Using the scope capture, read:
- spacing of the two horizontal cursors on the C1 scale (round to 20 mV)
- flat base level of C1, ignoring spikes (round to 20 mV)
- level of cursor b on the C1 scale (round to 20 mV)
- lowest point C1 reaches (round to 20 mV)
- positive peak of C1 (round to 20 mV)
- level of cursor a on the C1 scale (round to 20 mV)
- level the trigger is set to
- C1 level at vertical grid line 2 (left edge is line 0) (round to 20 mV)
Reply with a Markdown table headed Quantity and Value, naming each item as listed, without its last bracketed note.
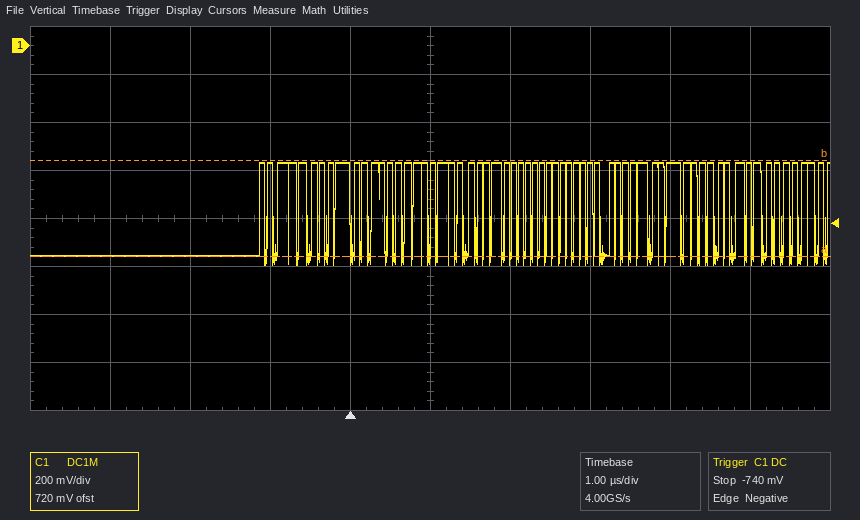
| Quantity | Value |
|---|---|
| spacing of the two horizontal cursors on the C1 scale | 400 mV |
| flat base level of C1, ignoring spikes | -880 mV |
| level of cursor b on the C1 scale | -480 mV |
| lowest point C1 reaches | -920 mV |
| positive peak of C1 | -480 mV |
| level of cursor a on the C1 scale | -880 mV |
| level the trigger is set to | -740 mV |
| C1 level at vertical grid line 2 (left edge is line 0) | -880 mV |
